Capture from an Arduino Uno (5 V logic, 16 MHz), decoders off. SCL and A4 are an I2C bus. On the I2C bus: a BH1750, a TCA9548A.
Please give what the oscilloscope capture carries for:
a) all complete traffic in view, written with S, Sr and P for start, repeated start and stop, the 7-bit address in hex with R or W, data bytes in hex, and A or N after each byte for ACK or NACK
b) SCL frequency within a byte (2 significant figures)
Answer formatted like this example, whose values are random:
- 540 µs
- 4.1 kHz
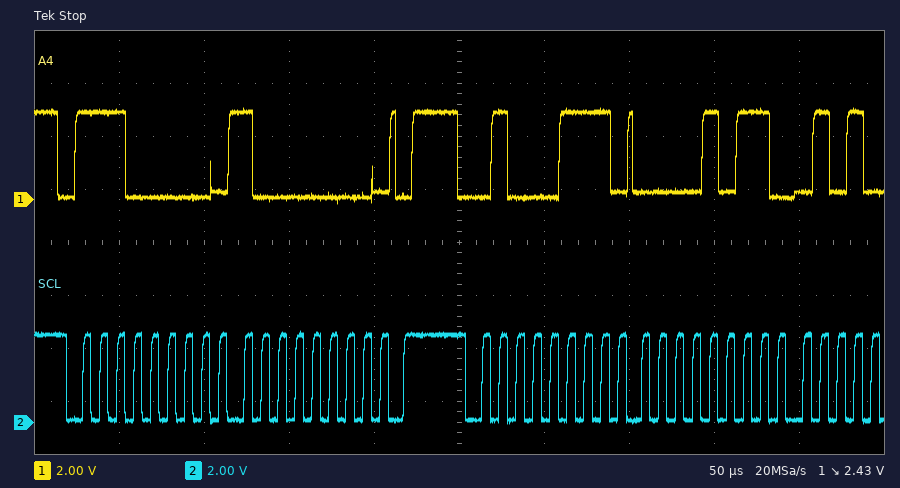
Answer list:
- S 70W A 80 A P S 23R A 0B A
- 100 kHz
